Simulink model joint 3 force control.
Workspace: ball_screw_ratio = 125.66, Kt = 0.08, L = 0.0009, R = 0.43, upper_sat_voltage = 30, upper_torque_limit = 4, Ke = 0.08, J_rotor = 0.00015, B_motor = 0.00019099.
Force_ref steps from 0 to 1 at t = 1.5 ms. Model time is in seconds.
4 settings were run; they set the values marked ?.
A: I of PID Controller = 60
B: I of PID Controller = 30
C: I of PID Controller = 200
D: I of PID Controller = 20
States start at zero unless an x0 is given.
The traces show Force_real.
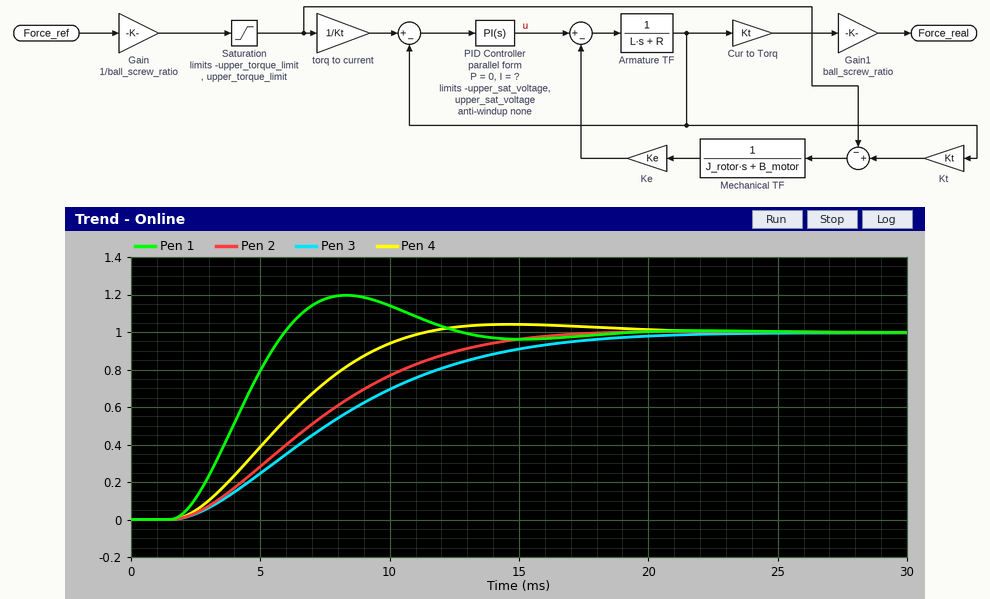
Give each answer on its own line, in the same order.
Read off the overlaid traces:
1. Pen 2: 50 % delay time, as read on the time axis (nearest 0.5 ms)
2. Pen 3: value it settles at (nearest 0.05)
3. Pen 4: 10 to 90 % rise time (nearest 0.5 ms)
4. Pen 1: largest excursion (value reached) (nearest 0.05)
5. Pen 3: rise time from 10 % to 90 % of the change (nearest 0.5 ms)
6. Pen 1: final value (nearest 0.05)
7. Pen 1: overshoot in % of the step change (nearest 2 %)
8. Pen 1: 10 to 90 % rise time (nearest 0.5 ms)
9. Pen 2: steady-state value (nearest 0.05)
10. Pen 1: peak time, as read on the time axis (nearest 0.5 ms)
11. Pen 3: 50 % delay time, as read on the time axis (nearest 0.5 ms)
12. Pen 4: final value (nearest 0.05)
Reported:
7.0 ms
1.00
6.5 ms
1.20
11.0 ms
1.00
20 %
3.0 ms
1.00
8.5 ms
7.5 ms
1.00
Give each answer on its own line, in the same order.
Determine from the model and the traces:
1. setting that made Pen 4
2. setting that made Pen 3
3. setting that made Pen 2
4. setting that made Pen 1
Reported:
A
D
B
C
